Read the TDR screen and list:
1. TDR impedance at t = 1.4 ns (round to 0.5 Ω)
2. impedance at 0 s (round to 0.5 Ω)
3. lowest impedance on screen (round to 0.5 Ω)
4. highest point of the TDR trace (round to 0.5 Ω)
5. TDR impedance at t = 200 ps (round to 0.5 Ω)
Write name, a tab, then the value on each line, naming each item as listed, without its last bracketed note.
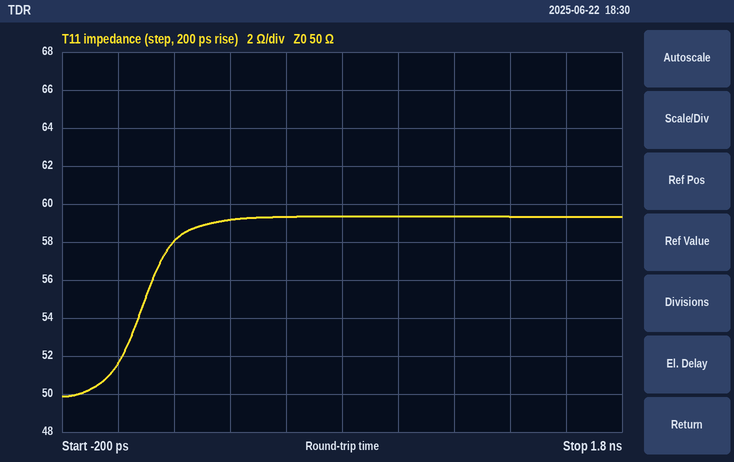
TDR impedance at t = 1.4 ns	59.5 Ω
impedance at 0 s	51.5 Ω
lowest impedance on screen	50.0 Ω
highest point of the TDR trace	59.5 Ω
TDR impedance at t = 200 ps	58.0 Ω
